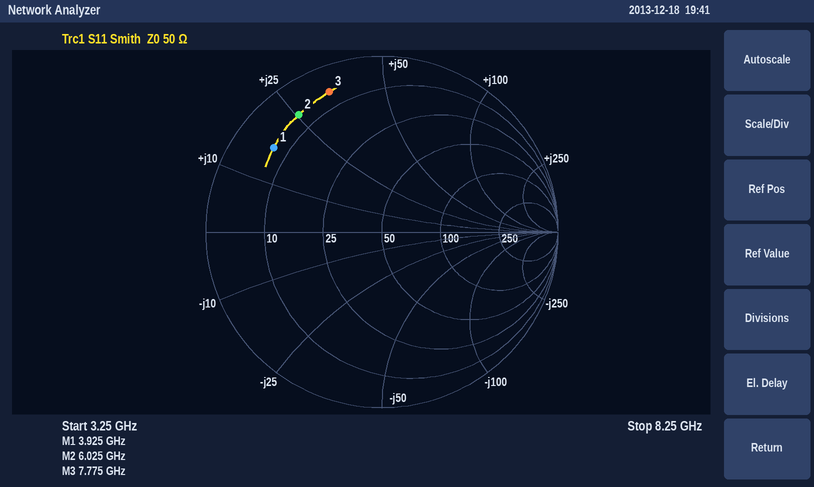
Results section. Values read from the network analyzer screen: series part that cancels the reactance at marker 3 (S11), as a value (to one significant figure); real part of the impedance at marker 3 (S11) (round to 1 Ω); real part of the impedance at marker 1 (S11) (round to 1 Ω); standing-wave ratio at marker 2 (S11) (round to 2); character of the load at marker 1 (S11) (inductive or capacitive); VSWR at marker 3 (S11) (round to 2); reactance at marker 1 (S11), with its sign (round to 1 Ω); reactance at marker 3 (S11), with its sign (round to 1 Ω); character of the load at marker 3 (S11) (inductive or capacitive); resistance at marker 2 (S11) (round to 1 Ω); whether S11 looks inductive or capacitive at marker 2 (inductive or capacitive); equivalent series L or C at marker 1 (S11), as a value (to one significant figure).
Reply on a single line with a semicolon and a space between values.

600 fF; 6 Ω; 7 Ω; 10; inductive; 12; +17 Ω; +34 Ω; inductive; 6 Ω; inductive; 700 pH
